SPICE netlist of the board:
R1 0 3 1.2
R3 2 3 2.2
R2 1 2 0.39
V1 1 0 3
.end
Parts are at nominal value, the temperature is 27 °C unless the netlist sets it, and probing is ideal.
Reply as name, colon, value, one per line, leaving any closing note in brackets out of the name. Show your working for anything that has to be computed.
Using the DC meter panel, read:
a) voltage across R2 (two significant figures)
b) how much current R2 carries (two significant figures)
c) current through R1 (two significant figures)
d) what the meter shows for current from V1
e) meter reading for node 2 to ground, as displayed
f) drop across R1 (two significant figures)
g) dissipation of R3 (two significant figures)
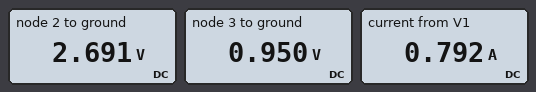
voltage across R2: 3 V - 2.691 V = 310 mV
how much current R2 carries: (3 V - 2.691 V) / 390 mΩ = 790 mA
current through R1: (950 mV) / 1.2 Ω = 790 mA
what the meter shows for current from V1: 0.792 A
meter reading for node 2 to ground, as displayed: 2.691 V
drop across R1: 950 mV = 950 mV
dissipation of R3: (2.691 V - 950 mV)^2 / 2.2 Ω = 1.4 W
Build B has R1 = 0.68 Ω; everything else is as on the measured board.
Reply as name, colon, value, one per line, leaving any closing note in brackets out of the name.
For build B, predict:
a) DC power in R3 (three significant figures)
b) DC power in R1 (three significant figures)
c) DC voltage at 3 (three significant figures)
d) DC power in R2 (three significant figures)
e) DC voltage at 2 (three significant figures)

DC power in R3: 1.85 W
DC power in R1: 572 mW
DC voltage at 3: 624 mV
DC power in R2: 328 mW
DC voltage at 2: 2.64 V
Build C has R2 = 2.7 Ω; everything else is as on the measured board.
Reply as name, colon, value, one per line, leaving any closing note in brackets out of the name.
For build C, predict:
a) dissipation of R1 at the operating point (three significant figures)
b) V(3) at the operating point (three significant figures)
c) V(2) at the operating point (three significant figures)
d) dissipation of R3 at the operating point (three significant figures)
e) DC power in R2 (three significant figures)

dissipation of R1 at the operating point: 290 mW
V(3) at the operating point: 590 mV
V(2) at the operating point: 1.67 V
dissipation of R3 at the operating point: 532 mW
DC power in R2: 653 mW
